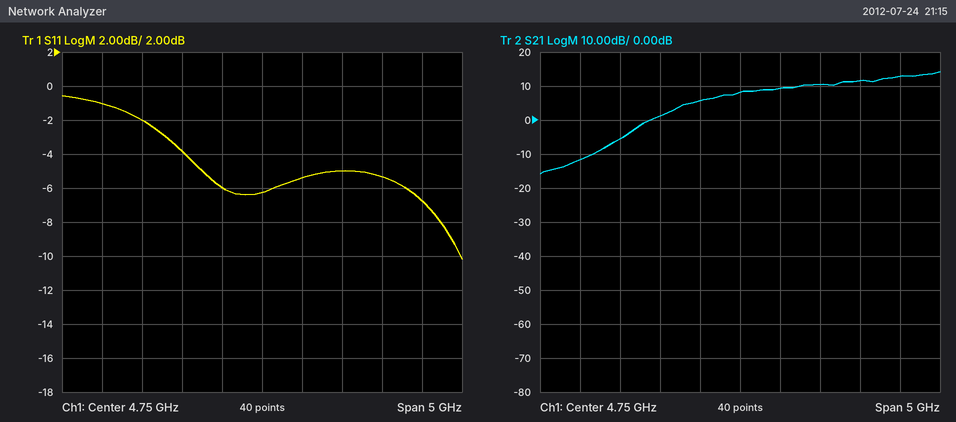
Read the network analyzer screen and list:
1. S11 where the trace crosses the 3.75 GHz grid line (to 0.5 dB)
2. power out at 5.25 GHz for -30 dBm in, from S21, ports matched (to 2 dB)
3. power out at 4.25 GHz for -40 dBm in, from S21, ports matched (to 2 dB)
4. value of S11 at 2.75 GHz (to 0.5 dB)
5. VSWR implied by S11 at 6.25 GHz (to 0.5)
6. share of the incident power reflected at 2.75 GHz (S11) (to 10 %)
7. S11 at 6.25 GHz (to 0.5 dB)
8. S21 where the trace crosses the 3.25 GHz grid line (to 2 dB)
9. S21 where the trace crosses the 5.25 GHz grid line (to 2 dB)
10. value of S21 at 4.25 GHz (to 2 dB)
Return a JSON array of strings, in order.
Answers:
["-4.0 dB", "-20 dBm", "-34 dBm", "-1.0 dB", "3.5", "80 %", "-5.5 dB", "-6 dB", "10 dB", "6 dB"]
